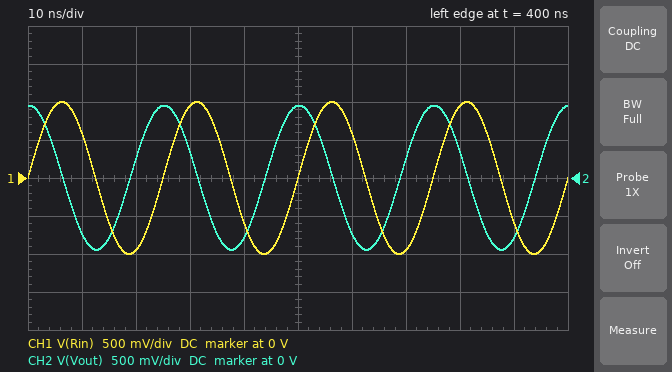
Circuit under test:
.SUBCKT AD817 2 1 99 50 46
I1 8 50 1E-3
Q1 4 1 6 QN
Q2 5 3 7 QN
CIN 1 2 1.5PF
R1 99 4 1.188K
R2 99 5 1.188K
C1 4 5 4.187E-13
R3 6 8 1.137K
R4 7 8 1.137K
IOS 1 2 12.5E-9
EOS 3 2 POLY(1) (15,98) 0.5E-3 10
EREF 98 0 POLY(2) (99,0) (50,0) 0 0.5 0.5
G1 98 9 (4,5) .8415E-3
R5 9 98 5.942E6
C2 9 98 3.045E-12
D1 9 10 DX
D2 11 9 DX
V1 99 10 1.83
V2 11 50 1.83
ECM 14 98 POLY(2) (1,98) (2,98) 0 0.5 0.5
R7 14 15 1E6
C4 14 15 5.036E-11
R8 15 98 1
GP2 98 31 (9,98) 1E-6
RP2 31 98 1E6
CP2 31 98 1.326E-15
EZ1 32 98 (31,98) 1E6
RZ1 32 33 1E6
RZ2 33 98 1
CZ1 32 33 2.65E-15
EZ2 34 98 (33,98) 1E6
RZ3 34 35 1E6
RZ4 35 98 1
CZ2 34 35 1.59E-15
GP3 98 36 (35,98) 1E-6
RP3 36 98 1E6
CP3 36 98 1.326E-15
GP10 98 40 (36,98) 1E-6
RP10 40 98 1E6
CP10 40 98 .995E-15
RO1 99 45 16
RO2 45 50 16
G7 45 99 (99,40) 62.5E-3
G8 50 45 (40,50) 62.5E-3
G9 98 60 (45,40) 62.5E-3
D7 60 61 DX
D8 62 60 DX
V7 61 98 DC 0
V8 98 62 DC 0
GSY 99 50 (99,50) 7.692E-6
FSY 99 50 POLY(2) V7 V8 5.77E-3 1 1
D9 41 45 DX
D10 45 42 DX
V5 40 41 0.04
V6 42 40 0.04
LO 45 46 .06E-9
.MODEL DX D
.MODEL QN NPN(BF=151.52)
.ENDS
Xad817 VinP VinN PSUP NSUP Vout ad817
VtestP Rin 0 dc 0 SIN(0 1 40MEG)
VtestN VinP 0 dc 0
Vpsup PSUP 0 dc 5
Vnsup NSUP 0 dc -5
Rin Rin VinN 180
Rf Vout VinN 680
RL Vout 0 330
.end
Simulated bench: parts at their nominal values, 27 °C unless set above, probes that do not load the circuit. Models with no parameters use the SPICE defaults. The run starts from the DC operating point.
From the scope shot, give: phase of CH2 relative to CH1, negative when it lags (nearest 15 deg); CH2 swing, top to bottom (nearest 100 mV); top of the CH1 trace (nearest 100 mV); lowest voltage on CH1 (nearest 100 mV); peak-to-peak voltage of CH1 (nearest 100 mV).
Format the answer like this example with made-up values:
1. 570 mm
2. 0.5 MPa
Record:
1. 90 deg
2. 1.9 V
3. 1.0 V
4. -1.0 V
5. 2.0 V
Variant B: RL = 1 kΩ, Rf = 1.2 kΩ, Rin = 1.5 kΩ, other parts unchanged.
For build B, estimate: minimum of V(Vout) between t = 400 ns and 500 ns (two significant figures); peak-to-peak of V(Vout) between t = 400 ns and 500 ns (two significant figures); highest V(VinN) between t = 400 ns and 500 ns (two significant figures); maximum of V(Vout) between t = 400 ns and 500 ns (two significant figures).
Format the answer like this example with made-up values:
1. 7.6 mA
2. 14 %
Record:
1. -560 mV
2. 1.1 V
3. 480 mV
4. 570 mV
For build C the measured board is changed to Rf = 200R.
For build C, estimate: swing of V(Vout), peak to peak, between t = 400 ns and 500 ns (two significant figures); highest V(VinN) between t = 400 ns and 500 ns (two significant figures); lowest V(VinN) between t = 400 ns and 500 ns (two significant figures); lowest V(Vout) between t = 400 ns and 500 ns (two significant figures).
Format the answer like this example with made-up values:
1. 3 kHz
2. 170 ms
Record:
1. 1.2 V
2. 530 mV
3. -530 mV
4. -600 mV
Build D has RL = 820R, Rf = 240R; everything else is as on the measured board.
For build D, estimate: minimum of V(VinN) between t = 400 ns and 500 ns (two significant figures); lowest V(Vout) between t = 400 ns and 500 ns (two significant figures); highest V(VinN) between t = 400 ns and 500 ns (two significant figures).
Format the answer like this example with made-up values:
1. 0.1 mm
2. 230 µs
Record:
1. -580 mV
2. -670 mV
3. 580 mV
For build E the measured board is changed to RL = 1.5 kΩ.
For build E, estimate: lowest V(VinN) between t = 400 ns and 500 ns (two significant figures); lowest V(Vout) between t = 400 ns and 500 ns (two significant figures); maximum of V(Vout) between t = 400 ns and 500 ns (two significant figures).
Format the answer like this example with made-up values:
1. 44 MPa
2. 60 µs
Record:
1. -820 mV
2. -960 mV
3. 970 mV
